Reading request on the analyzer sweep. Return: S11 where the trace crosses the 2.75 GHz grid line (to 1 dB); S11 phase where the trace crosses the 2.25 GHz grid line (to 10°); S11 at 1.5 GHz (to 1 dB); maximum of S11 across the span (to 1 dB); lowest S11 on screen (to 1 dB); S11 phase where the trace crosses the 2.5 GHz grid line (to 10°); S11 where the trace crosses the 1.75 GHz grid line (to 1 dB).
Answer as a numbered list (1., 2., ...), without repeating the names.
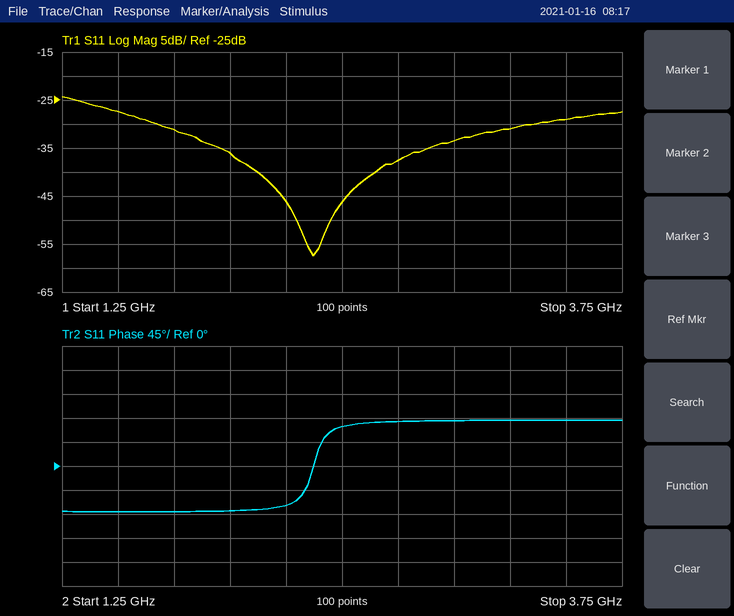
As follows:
1. -38 dB
2. -70°
3. -27 dB
4. -24 dB
5. -57 dB
6. 70°
7. -31 dB
